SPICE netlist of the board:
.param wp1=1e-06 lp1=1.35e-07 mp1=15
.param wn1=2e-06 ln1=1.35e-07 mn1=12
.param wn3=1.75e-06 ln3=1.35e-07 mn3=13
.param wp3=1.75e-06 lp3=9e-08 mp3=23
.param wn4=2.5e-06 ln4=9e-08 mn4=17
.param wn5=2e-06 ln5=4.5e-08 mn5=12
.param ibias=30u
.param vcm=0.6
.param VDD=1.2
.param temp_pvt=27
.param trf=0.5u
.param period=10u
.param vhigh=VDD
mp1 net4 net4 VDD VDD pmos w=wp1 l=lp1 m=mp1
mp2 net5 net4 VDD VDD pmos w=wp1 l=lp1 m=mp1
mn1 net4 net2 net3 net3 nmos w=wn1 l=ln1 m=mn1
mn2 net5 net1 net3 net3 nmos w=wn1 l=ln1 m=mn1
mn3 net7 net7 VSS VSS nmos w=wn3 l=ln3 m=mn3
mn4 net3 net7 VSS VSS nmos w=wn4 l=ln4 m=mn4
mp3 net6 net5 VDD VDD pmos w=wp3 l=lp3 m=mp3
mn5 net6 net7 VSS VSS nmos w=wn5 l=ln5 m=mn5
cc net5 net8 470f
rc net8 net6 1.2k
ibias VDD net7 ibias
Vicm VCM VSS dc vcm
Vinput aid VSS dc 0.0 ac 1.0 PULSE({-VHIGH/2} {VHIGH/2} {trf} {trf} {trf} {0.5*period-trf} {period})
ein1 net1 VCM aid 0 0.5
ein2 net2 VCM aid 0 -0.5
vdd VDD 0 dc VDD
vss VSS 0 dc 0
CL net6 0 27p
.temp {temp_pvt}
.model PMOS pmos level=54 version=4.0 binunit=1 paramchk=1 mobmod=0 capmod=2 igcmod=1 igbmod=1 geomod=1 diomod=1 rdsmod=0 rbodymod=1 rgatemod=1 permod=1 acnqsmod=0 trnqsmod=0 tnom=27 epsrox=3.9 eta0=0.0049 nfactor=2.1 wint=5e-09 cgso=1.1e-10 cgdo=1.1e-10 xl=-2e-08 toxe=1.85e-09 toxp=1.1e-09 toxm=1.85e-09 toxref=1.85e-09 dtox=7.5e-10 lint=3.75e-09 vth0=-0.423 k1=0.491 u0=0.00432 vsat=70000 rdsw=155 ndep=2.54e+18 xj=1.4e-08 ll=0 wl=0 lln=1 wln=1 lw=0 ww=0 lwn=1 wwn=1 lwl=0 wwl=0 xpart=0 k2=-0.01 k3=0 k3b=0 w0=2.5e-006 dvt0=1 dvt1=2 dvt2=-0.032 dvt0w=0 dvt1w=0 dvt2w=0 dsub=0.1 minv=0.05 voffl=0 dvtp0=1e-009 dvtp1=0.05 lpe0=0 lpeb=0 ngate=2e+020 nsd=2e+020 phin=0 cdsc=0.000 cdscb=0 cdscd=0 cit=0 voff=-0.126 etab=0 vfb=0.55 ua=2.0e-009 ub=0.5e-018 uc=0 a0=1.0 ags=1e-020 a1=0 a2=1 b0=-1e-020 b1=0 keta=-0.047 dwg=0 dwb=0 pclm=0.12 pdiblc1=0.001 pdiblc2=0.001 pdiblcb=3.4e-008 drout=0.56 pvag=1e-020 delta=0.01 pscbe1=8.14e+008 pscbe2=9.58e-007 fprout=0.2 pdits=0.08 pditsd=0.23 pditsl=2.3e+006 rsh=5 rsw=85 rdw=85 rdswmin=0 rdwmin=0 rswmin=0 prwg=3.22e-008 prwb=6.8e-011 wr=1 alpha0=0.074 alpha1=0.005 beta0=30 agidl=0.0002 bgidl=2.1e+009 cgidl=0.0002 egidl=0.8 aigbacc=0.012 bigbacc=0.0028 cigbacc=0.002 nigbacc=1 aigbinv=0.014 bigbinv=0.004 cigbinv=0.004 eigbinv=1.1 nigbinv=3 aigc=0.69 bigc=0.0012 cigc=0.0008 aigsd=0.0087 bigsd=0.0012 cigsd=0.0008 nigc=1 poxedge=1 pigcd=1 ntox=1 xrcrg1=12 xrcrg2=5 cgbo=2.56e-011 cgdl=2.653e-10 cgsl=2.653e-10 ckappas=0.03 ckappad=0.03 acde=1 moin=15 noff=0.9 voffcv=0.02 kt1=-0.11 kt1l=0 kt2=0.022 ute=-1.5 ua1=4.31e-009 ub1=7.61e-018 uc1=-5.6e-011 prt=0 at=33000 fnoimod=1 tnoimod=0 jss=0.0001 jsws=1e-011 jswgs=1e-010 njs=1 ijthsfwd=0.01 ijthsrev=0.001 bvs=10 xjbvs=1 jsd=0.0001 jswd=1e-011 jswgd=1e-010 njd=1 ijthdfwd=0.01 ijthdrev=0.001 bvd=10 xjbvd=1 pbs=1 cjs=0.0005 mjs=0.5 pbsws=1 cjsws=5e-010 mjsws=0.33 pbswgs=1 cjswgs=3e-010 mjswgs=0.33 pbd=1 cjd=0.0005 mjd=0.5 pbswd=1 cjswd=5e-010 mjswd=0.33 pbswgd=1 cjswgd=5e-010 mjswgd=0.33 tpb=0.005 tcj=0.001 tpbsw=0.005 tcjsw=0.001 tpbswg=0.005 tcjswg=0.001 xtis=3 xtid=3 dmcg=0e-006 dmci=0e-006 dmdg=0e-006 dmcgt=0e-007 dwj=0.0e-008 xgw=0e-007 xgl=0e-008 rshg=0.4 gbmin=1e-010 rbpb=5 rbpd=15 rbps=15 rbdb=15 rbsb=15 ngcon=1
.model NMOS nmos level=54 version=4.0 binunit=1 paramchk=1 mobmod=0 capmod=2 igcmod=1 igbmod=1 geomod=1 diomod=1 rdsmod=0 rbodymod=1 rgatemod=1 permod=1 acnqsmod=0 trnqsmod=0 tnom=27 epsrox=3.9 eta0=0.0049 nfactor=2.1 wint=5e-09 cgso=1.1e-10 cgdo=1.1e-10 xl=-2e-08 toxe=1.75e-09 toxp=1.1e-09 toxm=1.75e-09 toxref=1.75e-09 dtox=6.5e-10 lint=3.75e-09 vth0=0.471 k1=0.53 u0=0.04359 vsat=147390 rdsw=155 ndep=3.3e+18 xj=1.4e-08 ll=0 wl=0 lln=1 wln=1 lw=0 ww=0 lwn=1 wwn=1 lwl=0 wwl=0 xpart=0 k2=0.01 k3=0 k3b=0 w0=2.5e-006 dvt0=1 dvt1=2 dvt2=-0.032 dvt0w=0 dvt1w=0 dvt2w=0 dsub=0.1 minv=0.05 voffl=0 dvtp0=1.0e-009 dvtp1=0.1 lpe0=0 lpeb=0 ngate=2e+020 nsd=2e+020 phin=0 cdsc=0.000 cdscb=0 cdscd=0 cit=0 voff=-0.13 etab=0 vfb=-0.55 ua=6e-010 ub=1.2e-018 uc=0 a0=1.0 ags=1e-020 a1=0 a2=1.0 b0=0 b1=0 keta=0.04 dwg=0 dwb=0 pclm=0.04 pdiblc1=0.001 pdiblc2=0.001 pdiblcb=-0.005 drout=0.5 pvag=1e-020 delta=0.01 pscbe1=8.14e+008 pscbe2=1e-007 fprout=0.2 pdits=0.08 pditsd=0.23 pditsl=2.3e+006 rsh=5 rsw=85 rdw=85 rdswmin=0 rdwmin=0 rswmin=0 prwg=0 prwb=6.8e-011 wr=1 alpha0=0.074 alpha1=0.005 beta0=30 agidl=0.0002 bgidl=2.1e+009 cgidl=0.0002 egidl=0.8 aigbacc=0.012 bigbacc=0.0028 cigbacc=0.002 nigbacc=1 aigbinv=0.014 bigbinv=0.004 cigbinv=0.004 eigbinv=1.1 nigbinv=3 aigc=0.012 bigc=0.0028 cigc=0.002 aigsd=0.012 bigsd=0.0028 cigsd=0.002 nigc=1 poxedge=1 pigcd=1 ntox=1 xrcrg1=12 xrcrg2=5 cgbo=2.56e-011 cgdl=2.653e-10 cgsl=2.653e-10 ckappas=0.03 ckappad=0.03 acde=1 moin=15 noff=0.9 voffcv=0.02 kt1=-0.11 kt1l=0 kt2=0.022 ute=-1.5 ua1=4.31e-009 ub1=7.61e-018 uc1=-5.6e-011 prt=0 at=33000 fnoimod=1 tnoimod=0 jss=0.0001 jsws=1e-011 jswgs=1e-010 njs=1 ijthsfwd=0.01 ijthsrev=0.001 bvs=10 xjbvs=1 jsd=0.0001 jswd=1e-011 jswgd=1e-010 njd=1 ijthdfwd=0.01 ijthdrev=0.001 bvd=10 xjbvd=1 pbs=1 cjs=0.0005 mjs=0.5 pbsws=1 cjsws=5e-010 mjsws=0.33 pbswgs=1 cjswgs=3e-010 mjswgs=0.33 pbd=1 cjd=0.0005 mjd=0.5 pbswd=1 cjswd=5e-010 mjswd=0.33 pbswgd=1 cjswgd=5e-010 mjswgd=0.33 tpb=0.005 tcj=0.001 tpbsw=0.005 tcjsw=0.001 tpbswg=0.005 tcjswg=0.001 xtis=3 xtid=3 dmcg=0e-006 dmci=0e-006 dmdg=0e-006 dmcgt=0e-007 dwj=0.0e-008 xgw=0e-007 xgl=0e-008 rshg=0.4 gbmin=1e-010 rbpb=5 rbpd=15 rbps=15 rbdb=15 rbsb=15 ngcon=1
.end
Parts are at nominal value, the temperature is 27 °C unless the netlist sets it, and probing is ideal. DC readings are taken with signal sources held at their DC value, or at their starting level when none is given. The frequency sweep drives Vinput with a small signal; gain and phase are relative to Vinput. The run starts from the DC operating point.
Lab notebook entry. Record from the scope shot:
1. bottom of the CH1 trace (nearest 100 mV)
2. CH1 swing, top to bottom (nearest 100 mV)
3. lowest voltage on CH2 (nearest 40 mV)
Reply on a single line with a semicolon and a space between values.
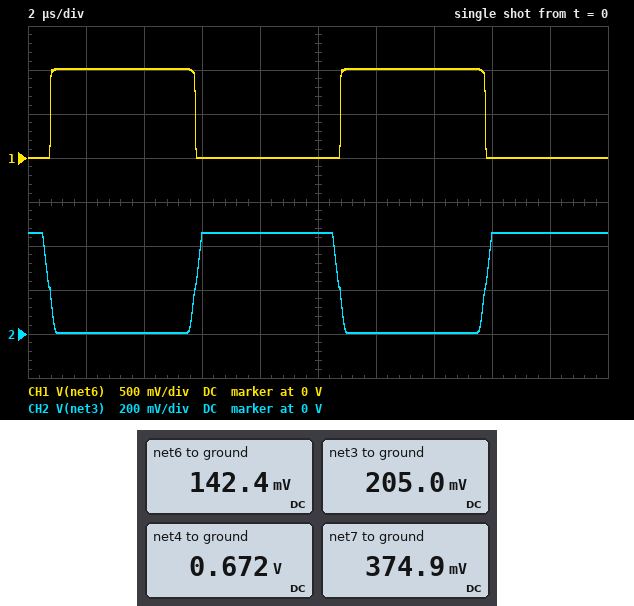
0 V; 1.0 V; 0 V
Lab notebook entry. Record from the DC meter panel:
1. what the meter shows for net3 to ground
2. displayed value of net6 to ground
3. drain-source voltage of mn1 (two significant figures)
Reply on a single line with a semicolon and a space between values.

205.0 mV; 142.4 mV; 470 mV
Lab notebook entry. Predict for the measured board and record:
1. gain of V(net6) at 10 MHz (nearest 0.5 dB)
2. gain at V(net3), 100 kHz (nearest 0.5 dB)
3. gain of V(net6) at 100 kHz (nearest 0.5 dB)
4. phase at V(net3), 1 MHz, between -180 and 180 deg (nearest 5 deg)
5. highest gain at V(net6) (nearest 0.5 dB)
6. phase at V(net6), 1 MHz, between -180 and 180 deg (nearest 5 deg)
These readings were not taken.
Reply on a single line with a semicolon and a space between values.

25.5 dB; -12.0 dB; 46.5 dB; 145 deg; 46.5 dB; -50 deg
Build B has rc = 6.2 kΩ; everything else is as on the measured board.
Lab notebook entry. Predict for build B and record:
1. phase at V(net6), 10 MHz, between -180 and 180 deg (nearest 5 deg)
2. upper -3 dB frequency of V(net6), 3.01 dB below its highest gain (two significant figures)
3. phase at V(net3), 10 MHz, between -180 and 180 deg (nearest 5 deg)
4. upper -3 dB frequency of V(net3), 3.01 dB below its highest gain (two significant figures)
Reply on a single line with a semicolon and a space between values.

-100 deg; 910 kHz; 150 deg; 960 kHz
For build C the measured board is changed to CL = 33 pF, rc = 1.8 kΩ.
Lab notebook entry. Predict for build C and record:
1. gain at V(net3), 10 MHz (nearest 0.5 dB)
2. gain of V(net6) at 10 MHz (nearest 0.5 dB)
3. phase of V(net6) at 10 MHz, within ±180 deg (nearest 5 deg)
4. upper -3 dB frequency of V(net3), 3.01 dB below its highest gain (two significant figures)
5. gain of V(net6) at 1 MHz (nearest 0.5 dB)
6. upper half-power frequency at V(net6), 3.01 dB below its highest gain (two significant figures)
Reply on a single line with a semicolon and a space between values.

-24.0 dB; 25.0 dB; -110 deg; 960 kHz; 43.0 dB; 900 kHz
